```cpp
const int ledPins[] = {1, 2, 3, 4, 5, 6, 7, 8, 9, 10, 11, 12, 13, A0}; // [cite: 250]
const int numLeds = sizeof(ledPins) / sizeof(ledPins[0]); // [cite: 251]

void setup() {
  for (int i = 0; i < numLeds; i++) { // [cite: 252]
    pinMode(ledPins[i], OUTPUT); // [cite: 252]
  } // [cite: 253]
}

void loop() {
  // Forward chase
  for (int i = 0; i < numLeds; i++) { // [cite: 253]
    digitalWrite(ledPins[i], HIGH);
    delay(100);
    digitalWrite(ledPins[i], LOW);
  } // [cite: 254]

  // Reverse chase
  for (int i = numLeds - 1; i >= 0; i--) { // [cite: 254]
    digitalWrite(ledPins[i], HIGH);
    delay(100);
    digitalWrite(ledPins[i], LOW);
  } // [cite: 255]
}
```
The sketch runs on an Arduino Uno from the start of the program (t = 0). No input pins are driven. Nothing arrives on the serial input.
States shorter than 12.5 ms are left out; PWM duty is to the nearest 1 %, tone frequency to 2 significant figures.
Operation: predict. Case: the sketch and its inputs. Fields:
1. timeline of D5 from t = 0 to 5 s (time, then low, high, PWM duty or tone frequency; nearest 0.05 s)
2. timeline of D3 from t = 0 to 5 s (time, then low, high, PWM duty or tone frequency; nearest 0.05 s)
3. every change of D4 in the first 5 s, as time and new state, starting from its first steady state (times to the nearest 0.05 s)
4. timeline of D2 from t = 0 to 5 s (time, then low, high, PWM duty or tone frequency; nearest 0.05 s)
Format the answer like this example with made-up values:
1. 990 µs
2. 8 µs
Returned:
1. 0 s low; 0.4 s high; 0.5 s low; 2.3 s high; 2.4 s low; 3.2 s high; 3.3 s low
2. 0 s low; 0.2 s high; 0.3 s low; 2.5 s high; 2.6 s low; 3 s high; 3.1 s low
3. 0 s low; 0.3 s high; 0.4 s low; 2.4 s high; 2.5 s low; 3.1 s high; 3.2 s low
4. 0 s low; 0.1 s high; 0.2 s low; 2.6 s high; 2.7 s low; 2.9 s high; 3 s low
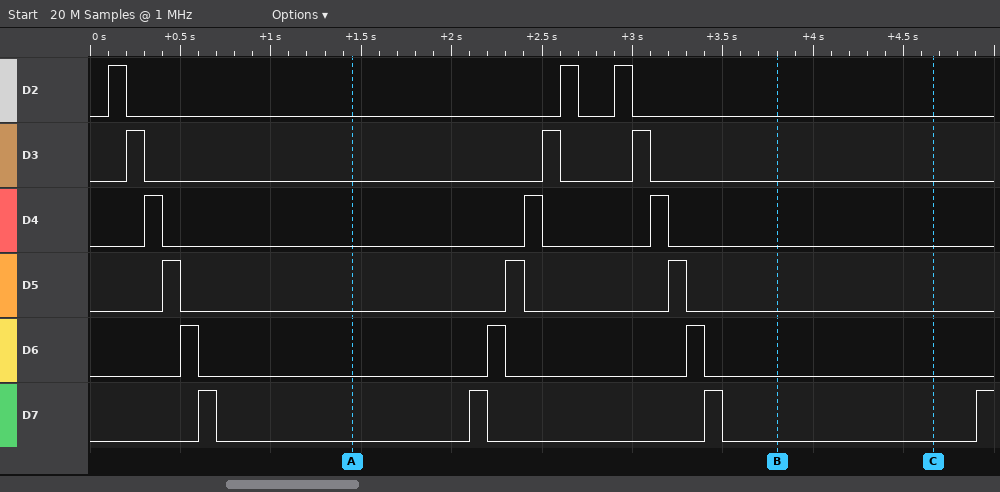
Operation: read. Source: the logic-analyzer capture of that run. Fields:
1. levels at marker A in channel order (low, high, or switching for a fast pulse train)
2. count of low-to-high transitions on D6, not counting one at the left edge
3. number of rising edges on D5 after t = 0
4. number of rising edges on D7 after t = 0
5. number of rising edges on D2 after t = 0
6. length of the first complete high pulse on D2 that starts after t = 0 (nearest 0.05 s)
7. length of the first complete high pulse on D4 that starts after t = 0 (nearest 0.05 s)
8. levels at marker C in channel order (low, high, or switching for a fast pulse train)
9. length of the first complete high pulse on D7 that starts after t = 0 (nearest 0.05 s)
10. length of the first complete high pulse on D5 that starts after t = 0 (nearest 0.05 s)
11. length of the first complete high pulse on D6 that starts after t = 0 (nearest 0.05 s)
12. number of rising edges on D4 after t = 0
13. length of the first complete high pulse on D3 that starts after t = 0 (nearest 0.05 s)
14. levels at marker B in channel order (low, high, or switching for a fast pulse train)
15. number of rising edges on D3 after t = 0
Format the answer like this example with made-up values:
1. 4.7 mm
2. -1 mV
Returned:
1. D2 low, D3 low, D4 low, D5 low, D6 low, D7 low
2. 3
3. 3
4. 4
5. 3
6. 0.10 s
7. 0.10 s
8. D2 low, D3 low, D4 low, D5 low, D6 low, D7 low
9. 0.10 s
10. 0.10 s
11. 0.10 s
12. 3
13. 0.10 s
14. D2 low, D3 low, D4 low, D5 low, D6 low, D7 low
15. 3
